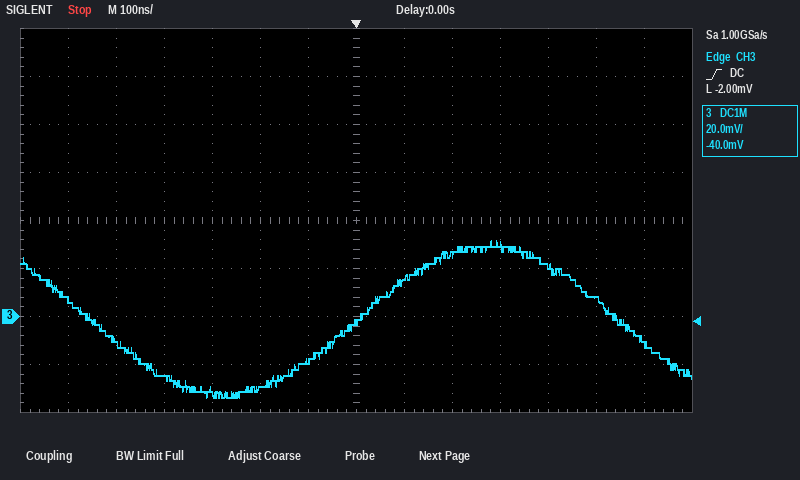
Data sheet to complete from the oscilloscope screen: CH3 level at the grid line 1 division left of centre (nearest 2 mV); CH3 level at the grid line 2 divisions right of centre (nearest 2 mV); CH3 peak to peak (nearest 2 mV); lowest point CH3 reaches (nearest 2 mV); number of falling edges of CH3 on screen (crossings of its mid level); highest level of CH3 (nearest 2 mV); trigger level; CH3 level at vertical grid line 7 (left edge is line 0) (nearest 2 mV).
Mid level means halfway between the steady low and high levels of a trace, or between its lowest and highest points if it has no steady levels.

-18 mV
26 mV
66 mV
-34 mV
2
32 mV
-2.00 mV
-2 mV
